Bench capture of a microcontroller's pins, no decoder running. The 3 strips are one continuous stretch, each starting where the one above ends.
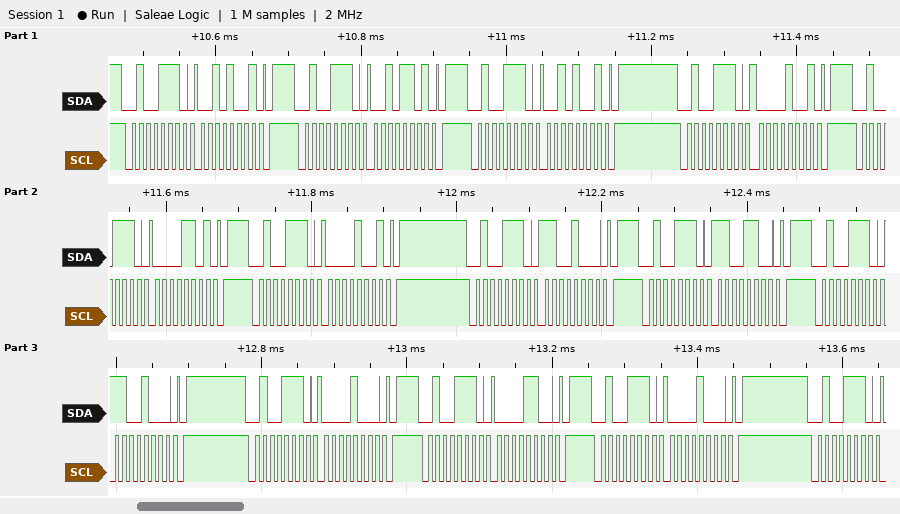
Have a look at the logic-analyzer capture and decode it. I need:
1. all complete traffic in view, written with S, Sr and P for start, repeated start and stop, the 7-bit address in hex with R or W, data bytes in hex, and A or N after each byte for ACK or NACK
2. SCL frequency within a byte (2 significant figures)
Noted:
S 27W A 29 A P S 27W A 2D A P S 27W A 29 A P S 27W A 09 A P S 27W A 0D A P S 27W A 09 A P S 27W A C8 A P S 27W A CC A P S 27W A C8 A P S 27W A 08 A P S 27W A 0C A P S 27W A 08 A P S 27W A
100 kHz
